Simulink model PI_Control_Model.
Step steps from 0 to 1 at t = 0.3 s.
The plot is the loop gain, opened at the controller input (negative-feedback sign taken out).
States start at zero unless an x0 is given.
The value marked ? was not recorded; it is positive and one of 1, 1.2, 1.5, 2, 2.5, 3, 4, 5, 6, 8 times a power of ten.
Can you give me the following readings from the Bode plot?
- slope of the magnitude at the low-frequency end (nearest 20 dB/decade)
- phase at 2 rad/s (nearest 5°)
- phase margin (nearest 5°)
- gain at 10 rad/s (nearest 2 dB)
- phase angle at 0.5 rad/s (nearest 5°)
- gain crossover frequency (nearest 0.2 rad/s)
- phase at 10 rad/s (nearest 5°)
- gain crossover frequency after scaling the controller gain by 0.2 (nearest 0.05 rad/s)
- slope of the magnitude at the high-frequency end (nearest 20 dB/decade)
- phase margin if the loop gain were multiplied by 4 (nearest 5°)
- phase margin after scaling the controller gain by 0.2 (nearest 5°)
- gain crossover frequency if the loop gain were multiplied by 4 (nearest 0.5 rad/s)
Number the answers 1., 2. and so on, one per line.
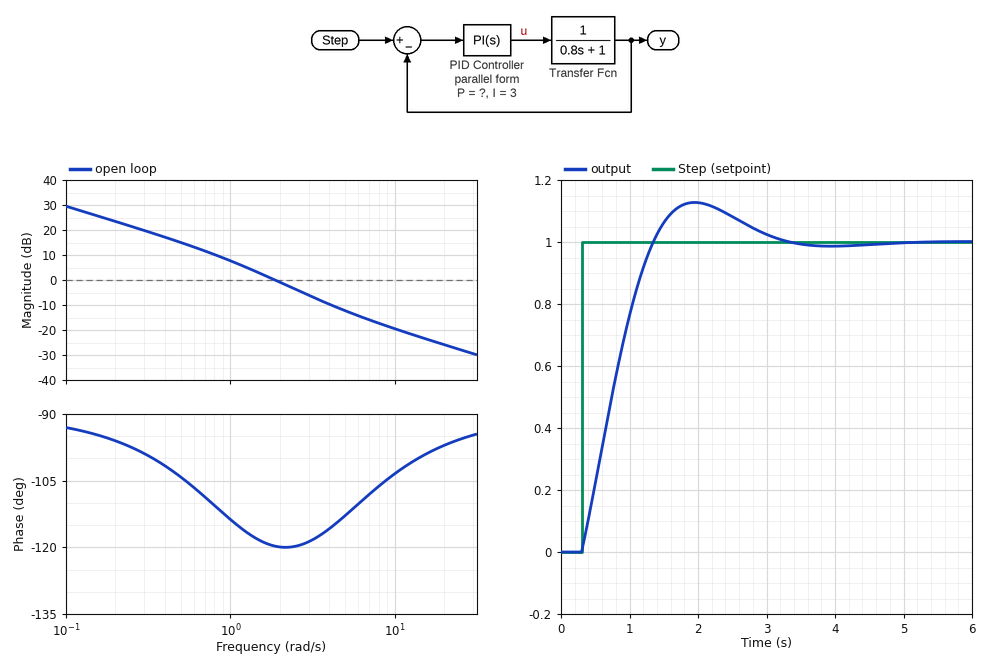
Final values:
1. -20 dB/decade
2. -120°
3. 60°
4. -20 dB
5. -105°
6. 1.8 rad/s
7. -105°
8. 0.55 rad/s
9. -20 dB/decade
10. 65°
11. 75°
12. 5.0 rad/s
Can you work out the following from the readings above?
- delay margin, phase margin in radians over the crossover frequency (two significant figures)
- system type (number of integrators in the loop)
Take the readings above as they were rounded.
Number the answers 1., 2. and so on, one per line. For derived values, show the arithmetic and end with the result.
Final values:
1. 60 × π / 180 / 1.8 = 0.58 s
2. 1
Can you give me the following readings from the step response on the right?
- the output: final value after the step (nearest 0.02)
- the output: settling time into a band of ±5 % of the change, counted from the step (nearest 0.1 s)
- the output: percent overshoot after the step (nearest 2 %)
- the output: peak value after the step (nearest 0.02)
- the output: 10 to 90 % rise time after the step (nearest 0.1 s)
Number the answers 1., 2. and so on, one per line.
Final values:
1. 1.00
2. 2.5 s
3. 12 %
4. 1.12
5. 0.8 s
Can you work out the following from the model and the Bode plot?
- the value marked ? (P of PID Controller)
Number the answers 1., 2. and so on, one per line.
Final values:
1. 0.8
